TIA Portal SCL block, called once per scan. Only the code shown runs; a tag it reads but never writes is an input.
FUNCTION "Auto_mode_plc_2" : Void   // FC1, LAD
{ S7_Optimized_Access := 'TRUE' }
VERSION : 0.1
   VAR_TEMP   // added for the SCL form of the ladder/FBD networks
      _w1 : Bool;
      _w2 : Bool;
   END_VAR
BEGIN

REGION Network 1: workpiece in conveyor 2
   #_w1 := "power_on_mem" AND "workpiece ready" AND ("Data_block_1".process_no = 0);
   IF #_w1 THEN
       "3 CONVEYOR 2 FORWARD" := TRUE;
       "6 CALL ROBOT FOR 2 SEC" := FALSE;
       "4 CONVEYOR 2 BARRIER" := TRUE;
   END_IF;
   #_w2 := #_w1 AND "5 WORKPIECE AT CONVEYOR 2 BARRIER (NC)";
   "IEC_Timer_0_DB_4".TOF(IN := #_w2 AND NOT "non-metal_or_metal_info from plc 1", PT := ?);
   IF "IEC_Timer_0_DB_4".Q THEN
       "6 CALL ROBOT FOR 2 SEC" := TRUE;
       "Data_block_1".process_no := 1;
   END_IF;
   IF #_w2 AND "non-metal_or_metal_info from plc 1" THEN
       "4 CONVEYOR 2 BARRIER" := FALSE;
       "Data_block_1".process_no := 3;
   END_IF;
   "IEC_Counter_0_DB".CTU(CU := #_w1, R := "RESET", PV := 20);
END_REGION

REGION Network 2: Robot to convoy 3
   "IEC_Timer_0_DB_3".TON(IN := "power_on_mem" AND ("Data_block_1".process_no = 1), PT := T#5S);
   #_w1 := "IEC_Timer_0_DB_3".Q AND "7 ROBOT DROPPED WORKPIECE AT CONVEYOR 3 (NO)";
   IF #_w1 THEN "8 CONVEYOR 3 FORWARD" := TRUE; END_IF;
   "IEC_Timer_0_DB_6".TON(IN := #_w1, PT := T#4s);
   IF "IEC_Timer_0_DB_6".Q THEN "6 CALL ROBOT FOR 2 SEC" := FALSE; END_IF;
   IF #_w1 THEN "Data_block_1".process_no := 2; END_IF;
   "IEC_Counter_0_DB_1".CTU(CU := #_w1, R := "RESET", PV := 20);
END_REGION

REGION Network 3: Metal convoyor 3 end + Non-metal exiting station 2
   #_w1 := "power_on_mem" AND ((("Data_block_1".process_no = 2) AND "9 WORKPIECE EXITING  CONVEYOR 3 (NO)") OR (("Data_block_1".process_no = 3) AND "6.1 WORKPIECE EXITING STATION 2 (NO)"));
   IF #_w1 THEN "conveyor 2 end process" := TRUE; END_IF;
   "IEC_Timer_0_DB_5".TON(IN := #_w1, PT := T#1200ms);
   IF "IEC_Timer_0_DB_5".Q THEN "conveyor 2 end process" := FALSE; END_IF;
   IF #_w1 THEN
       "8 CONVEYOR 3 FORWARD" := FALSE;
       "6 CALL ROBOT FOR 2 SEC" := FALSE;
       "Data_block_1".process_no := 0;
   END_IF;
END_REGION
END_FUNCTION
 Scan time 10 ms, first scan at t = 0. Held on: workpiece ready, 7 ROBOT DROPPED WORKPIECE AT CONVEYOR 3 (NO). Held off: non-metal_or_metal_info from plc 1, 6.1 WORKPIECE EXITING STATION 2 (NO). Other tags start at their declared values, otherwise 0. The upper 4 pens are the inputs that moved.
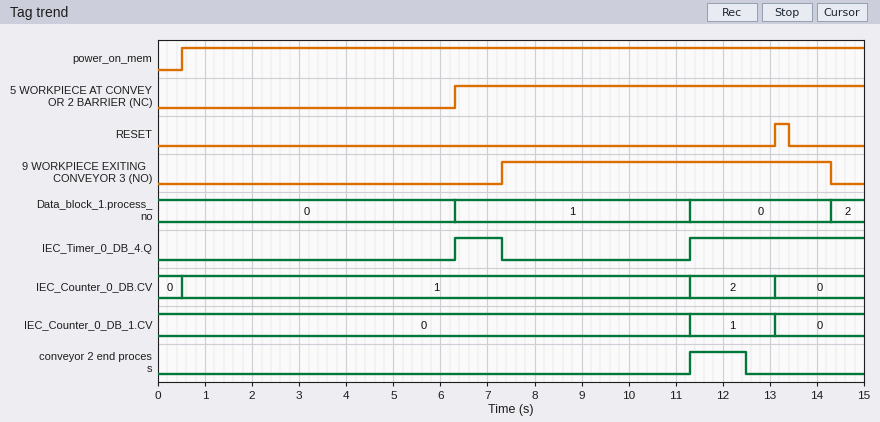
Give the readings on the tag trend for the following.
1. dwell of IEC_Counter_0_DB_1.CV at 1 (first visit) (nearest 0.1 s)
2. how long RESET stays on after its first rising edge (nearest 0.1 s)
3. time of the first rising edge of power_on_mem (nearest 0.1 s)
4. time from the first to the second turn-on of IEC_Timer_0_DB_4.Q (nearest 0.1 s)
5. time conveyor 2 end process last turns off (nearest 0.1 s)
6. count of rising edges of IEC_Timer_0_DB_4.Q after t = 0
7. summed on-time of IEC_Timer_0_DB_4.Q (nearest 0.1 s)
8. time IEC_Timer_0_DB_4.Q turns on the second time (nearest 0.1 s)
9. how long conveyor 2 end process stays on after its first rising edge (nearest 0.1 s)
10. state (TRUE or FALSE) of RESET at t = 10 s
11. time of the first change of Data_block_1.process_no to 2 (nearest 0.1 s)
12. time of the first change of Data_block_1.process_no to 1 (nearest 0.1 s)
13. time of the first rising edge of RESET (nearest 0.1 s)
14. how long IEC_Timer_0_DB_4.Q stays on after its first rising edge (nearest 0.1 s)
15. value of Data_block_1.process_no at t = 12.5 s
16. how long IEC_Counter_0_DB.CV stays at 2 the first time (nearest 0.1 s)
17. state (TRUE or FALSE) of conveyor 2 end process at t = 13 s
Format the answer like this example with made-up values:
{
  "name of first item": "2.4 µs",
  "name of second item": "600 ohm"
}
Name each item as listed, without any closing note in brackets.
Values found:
{
  "dwell of IEC_Counter_0_DB_1.CV at 1 (first visit)": "1.8 s",
  "how long RESET stays on after its first rising edge": "0.3 s",
  "time of the first rising edge of power_on_mem": "0.5 s",
  "time from the first to the second turn-on of IEC_Timer_0_DB_4.Q": "5.0 s",
  "time conveyor 2 end process last turns off": "12.5 s",
  "count of rising edges of IEC_Timer_0_DB_4.Q after t = 0": "2",
  "summed on-time of IEC_Timer_0_DB_4.Q": "4.7 s",
  "time IEC_Timer_0_DB_4.Q turns on the second time": "11.3 s",
  "how long conveyor 2 end process stays on after its first rising edge": "1.2 s",
  "state (TRUE or FALSE) of RESET at t = 10 s": "FALSE",
  "time of the first change of Data_block_1.process_no to 2": "14.3 s",
  "time of the first change of Data_block_1.process_no to 1": "6.3 s",
  "time of the first rising edge of RESET": "13.1 s",
  "how long IEC_Timer_0_DB_4.Q stays on after its first rising edge": "1.0 s",
  "value of Data_block_1.process_no at t = 12.5 s": "0",
  "how long IEC_Counter_0_DB.CV stays at 2 the first time": "1.8 s",
  "state (TRUE or FALSE) of conveyor 2 end process at t = 13 s": "FALSE"
}
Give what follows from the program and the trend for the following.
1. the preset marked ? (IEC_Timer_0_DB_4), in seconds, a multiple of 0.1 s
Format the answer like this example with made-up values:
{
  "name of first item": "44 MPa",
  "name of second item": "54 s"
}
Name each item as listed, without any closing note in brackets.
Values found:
{
  "the preset marked ? (IEC_Timer_0_DB_4), in seconds, a multiple of 0.1 s": "1.0 s"
}
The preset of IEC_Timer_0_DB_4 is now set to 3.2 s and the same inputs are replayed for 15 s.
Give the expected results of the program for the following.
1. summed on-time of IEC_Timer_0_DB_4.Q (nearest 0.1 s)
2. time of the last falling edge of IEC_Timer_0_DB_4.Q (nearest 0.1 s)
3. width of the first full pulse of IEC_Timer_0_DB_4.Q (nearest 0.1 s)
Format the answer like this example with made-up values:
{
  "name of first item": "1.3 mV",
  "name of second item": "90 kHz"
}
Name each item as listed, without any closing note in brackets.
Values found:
{
  "summed on-time of IEC_Timer_0_DB_4.Q": "6.9 s",
  "time of the last falling edge of IEC_Timer_0_DB_4.Q": "9.5 s",
  "width of the first full pulse of IEC_Timer_0_DB_4.Q": "3.2 s"
}
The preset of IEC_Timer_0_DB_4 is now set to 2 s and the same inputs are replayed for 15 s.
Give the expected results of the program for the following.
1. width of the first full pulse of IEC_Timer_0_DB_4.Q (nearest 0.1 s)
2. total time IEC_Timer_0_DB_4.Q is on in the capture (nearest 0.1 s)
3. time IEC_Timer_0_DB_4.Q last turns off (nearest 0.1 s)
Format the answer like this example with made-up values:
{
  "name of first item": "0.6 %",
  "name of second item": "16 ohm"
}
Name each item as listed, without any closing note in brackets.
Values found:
{
  "width of the first full pulse of IEC_Timer_0_DB_4.Q": "2.0 s",
  "total time IEC_Timer_0_DB_4.Q is on in the capture": "5.7 s",
  "time IEC_Timer_0_DB_4.Q last turns off": "8.3 s"
}
